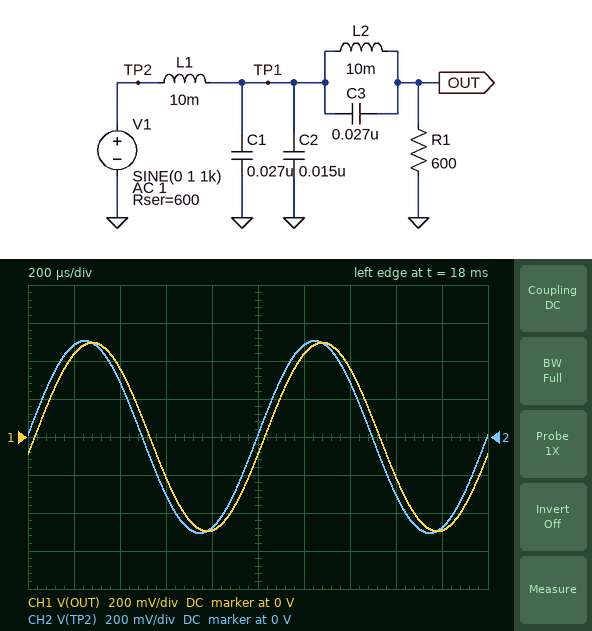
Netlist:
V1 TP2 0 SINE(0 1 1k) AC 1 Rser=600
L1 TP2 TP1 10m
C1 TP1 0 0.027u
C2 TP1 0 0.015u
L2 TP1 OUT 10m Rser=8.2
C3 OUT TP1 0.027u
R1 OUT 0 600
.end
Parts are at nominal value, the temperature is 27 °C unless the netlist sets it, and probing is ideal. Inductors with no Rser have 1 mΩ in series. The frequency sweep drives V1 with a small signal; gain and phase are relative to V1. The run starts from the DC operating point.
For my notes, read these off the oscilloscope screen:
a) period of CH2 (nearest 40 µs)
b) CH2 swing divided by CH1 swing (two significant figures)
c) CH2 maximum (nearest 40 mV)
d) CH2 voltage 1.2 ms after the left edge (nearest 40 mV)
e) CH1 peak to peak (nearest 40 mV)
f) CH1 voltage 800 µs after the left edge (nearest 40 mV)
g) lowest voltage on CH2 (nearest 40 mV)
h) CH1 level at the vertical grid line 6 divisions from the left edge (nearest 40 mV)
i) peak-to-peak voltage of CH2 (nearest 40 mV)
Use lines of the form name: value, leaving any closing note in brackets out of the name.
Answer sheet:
period of CH2: 1.00 ms
CH2 swing divided by CH1 swing: 1.0
CH2 maximum: 520 mV
CH2 voltage 1.2 ms after the left edge: 480 mV
CH1 peak to peak: 1.00 V
CH1 voltage 800 µs after the left edge: -480 mV
lowest voltage on CH2: -520 mV
CH1 level at the vertical grid line 6 divisions from the left edge: 440 mV
peak-to-peak voltage of CH2: 1.00 V
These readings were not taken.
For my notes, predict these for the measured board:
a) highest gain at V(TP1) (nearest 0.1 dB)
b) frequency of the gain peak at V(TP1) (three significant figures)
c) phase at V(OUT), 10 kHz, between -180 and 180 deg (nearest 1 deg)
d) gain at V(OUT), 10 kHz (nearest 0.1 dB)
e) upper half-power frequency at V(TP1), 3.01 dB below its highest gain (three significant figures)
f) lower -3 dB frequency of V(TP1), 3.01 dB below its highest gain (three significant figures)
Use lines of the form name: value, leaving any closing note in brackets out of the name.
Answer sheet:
highest gain at V(TP1): -0.9 dB
frequency of the gain peak at V(TP1): 7.86 kHz
phase at V(OUT), 10 kHz, between -180 and 180 deg: -38 deg
gain at V(OUT), 10 kHz: -29.1 dB
upper half-power frequency at V(TP1), 3.01 dB below its highest gain: 9.56 kHz
lower -3 dB frequency of V(TP1), 3.01 dB below its highest gain: 5.29 kHz
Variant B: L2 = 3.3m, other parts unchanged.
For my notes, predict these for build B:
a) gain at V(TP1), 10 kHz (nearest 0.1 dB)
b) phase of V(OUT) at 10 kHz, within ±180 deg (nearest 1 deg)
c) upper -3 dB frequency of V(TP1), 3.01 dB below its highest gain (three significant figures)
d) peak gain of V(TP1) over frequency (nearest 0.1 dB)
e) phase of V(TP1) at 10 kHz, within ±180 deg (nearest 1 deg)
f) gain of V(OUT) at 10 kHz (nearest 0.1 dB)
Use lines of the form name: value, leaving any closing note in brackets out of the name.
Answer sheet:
gain at V(TP1), 10 kHz: -6.3 dB
phase of V(OUT) at 10 kHz, within ±180 deg: -103 deg
upper -3 dB frequency of V(TP1), 3.01 dB below its highest gain: 14.4 kHz
peak gain of V(TP1) over frequency: -5.9 dB
phase of V(TP1) at 10 kHz, within ±180 deg: -75 deg
gain of V(OUT) at 10 kHz: -7.6 dB
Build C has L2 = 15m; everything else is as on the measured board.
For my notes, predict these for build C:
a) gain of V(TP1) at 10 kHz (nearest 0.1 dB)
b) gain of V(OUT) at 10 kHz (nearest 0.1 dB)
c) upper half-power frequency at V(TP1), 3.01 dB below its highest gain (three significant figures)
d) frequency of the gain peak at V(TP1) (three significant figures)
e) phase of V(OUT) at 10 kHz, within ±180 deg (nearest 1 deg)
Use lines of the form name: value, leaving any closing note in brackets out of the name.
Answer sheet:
gain of V(TP1) at 10 kHz: -7.0 dB
gain of V(OUT) at 10 kHz: -16.0 dB
upper half-power frequency at V(TP1), 3.01 dB below its highest gain: 8.31 kHz
frequency of the gain peak at V(TP1): 6.64 kHz
phase of V(OUT) at 10 kHz, within ±180 deg: -45 deg
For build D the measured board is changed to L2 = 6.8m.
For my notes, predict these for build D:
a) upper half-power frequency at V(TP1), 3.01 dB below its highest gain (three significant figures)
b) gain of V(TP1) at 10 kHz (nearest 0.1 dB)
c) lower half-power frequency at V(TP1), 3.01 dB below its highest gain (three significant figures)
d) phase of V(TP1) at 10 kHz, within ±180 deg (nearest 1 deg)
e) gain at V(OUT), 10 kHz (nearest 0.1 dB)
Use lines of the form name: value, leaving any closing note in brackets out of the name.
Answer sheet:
upper half-power frequency at V(TP1), 3.01 dB below its highest gain: 11.1 kHz
gain of V(TP1) at 10 kHz: -3.1 dB
lower half-power frequency at V(TP1), 3.01 dB below its highest gain: 4.27 kHz
phase of V(TP1) at 10 kHz, within ±180 deg: -97 deg
gain at V(OUT), 10 kHz: -12.1 dB
